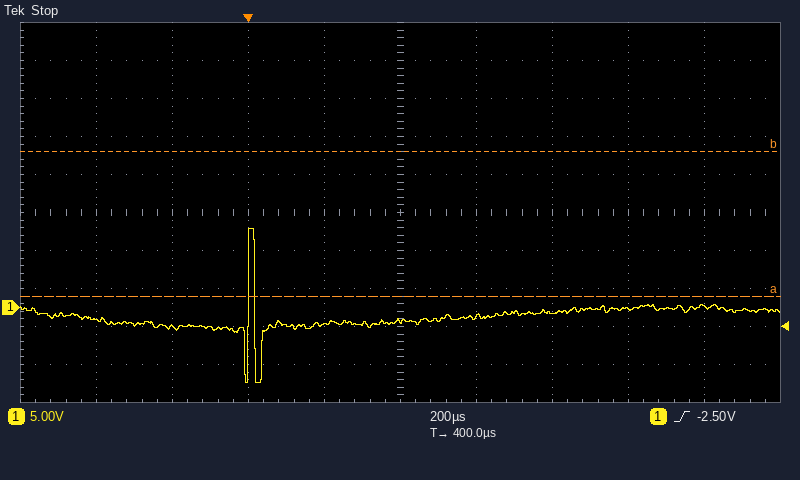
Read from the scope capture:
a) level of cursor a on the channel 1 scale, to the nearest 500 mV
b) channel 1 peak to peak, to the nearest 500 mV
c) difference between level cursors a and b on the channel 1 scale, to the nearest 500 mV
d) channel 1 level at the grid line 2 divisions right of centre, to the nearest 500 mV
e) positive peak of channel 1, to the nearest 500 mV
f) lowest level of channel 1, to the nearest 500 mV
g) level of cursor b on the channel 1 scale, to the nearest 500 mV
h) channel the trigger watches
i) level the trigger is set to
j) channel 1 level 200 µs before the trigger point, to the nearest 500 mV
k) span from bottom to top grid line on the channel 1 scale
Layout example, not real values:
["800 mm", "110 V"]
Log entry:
["1.5 V", "20.5 V", "19.0 V", "-500 mV", "10.5 V", "-10.0 V", "20.5 V", "channel 1", "-2.50 V", "-2.5 V", "50 V"]
